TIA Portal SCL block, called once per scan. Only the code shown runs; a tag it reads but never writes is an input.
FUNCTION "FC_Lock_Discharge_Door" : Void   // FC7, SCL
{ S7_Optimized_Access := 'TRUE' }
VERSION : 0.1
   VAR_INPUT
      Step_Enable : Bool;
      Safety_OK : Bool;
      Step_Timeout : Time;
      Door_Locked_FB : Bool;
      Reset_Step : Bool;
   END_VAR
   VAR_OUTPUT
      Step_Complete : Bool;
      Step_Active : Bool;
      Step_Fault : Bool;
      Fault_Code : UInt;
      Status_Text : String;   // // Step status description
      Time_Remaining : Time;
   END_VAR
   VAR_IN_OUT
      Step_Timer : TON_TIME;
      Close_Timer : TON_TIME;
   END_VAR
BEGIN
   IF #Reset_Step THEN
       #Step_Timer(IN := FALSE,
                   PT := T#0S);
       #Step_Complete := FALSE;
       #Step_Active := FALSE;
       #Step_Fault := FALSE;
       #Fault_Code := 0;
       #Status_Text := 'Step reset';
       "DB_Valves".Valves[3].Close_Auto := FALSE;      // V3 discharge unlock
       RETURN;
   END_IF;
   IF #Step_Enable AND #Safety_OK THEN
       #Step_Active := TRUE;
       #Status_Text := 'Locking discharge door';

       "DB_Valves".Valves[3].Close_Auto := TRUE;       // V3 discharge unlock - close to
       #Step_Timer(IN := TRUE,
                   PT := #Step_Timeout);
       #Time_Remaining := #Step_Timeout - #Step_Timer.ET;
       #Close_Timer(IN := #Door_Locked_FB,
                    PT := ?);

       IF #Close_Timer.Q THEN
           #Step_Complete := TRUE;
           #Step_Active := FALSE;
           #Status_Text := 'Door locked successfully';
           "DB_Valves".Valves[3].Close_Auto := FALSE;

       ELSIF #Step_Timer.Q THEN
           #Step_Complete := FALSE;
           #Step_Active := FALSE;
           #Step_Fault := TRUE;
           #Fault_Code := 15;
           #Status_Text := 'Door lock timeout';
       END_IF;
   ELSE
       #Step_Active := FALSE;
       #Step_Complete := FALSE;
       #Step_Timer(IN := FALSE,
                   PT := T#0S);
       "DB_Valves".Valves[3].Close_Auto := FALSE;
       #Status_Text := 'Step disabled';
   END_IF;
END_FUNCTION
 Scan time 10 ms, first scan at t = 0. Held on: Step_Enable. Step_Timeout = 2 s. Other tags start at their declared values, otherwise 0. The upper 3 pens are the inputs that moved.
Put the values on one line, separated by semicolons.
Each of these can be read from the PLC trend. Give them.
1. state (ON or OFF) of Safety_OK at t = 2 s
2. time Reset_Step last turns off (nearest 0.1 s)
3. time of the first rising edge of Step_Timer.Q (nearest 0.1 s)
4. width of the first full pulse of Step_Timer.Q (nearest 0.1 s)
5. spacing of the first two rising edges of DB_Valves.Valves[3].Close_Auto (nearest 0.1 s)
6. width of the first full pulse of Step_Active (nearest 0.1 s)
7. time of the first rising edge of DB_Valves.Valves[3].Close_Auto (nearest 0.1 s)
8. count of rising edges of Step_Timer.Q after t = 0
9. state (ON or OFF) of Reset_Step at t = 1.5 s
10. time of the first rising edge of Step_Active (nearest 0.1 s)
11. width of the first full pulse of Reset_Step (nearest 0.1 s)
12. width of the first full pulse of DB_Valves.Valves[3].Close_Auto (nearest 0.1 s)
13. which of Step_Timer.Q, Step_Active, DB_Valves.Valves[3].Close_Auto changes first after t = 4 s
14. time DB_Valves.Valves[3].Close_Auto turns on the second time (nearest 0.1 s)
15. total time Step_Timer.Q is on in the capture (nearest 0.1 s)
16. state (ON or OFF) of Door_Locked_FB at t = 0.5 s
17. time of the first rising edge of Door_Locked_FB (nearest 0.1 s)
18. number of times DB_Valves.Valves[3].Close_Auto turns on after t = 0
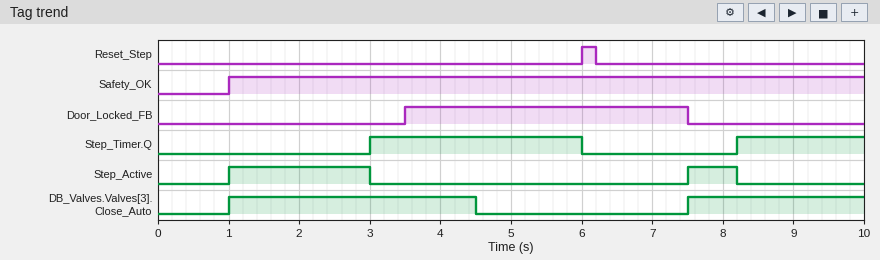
ON; 6.2 s; 3.0 s; 3.0 s; 6.5 s; 2.0 s; 1.0 s; 2; OFF; 1.0 s; 0.2 s; 3.5 s; DB_Valves.Valves[3].Close_Auto; 7.5 s; 4.8 s; OFF; 3.5 s; 2
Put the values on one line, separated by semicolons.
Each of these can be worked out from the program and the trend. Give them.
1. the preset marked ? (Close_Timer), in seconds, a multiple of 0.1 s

1.0 s
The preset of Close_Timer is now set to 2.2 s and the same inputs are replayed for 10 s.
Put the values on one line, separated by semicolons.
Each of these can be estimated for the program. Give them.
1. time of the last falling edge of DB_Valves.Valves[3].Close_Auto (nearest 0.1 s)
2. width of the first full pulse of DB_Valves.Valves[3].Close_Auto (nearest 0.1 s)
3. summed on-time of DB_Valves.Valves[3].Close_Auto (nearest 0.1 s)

5.7 s; 4.7 s; 7.2 s
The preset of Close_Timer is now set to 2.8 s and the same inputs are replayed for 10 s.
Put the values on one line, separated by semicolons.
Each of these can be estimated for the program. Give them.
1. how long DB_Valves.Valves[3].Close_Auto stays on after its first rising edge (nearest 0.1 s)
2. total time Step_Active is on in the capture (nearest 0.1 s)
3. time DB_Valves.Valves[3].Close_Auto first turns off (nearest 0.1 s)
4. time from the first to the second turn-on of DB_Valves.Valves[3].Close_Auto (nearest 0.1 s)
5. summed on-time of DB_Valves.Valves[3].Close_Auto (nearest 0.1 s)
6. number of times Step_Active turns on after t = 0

5.0 s; 2.8 s; 6.0 s; 5.2 s; 7.6 s; 3
